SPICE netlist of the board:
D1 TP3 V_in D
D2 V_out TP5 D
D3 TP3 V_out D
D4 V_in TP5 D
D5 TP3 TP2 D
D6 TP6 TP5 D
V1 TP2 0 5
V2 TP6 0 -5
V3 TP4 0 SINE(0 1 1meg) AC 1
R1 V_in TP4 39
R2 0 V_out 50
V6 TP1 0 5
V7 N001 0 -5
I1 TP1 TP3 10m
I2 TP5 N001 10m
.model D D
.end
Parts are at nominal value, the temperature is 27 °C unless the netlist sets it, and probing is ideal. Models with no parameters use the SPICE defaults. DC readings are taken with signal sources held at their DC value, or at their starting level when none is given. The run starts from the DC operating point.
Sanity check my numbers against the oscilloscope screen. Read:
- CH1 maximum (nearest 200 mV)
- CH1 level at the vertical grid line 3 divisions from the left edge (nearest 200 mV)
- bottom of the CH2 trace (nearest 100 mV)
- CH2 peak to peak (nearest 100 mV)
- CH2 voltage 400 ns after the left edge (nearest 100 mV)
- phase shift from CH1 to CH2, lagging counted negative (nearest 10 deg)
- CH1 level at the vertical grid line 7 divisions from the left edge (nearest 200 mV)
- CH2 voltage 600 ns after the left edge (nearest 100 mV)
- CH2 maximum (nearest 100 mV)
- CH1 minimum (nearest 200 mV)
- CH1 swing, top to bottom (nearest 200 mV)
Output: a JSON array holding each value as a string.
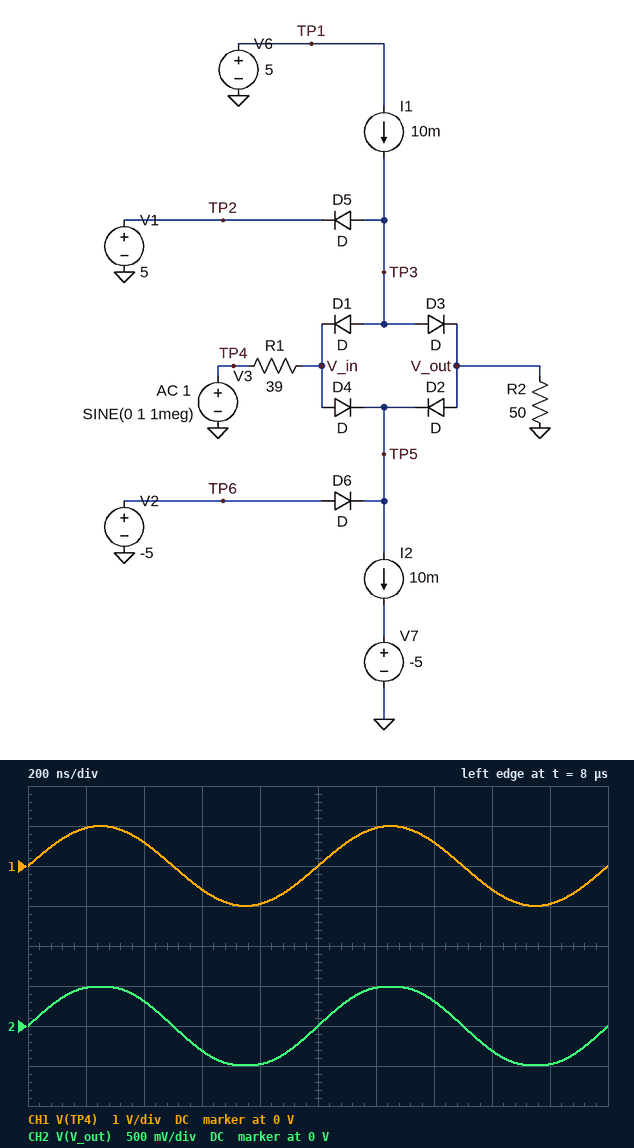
["1.0 V", "-600 mV", "-500 mV", "1.0 V", "300 mV", "0 deg", "600 mV", "-300 mV", "500 mV", "-1.0 V", "2.0 V"]
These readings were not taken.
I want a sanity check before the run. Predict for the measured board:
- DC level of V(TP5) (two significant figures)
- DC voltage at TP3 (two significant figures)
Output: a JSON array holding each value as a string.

["-700 mV", "700 mV"]
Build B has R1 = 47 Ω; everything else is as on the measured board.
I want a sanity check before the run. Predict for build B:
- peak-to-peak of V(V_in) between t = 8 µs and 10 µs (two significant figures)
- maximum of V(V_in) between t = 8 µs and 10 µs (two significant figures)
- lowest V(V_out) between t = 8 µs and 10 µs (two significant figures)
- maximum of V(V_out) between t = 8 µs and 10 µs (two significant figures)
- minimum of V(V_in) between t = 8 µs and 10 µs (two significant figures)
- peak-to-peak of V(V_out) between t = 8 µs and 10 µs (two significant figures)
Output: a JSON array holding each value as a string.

["1.1 V", "560 mV", "-470 mV", "470 mV", "-560 mV", "940 mV"]
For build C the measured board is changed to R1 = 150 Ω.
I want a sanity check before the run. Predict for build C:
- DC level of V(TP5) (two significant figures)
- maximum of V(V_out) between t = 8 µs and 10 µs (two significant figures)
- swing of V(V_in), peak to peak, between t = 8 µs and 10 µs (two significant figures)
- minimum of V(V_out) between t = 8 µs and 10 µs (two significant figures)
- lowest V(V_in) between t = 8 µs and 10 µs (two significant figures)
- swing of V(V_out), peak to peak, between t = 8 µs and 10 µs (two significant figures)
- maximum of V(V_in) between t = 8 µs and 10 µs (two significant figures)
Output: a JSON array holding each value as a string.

["-700 mV", "240 mV", "540 mV", "-240 mV", "-270 mV", "490 mV", "270 mV"]
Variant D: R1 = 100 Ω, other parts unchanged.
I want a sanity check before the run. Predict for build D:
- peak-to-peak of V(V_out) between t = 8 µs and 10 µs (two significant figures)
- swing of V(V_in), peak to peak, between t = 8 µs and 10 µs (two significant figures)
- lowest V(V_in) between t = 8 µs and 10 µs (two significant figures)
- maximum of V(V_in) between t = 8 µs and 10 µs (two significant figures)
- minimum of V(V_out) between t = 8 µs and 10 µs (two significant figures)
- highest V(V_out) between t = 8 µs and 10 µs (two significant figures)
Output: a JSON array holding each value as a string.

["640 mV", "720 mV", "-360 mV", "360 mV", "-320 mV", "320 mV"]
